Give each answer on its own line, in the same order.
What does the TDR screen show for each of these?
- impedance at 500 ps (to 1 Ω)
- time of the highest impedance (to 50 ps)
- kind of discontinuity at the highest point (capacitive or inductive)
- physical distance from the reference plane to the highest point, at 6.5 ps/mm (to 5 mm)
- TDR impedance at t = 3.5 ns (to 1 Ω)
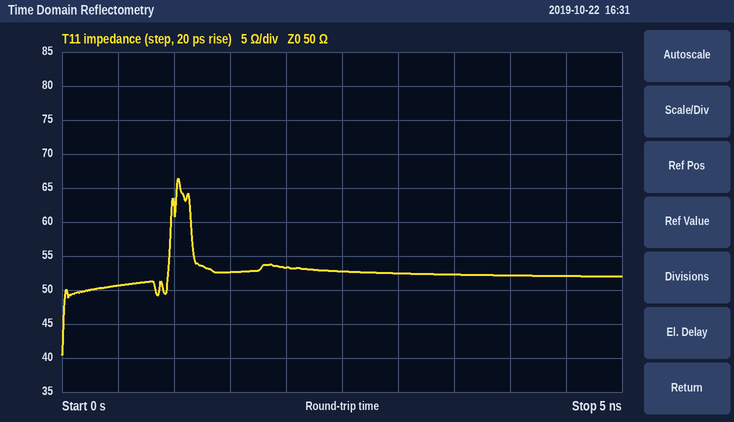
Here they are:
51 Ω
1.05 ns
inductive
80 mm
52 Ω
